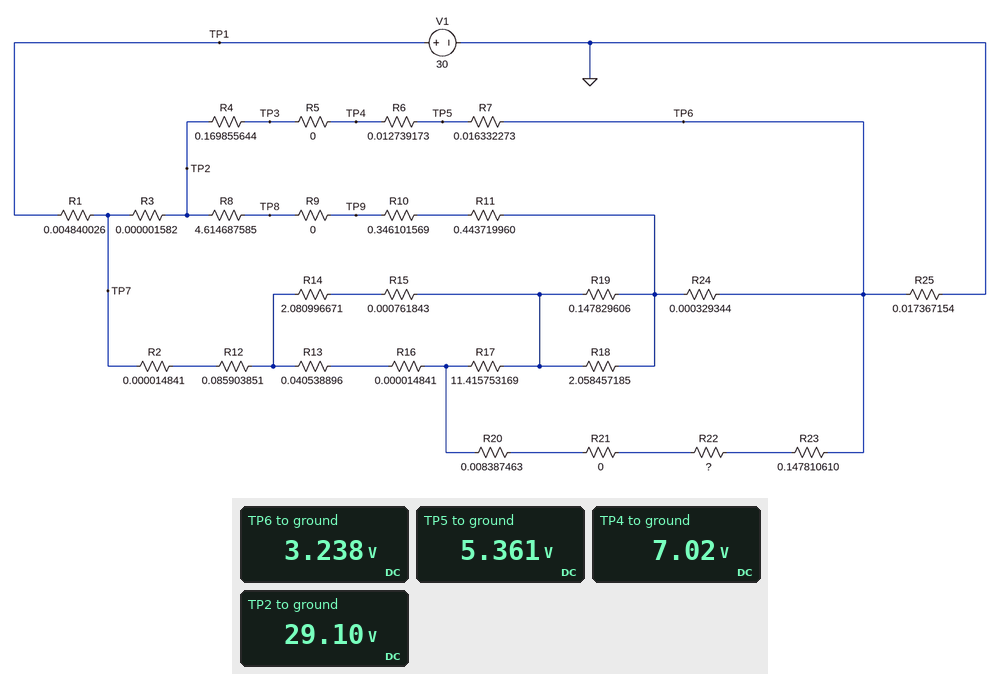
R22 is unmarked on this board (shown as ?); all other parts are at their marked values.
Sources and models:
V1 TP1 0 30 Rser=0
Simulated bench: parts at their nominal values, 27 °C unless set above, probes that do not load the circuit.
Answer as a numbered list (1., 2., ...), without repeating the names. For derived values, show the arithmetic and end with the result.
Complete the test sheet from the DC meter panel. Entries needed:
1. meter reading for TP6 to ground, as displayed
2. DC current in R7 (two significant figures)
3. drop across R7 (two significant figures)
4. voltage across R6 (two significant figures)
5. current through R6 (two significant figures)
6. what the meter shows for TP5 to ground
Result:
1. 3.238 V
2. (5.361 V - 3.238 V) / 16.33 mΩ = 130 A
3. 5.361 V - 3.238 V = 2.1 V
4. 7.02 V - 5.361 V = 1.7 V
5. (7.02 V - 5.361 V) / 12.74 mΩ = 130 A
6. 5.361 V
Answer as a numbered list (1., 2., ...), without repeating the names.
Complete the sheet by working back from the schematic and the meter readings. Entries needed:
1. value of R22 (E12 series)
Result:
1. 0.33 Ω
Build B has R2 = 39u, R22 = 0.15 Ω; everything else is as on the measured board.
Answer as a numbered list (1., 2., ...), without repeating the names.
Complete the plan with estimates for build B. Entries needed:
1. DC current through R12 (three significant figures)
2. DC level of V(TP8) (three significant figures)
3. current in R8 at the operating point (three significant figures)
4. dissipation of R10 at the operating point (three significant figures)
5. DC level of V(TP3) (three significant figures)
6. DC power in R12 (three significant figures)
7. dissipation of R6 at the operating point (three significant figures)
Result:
1. 67.1 A
2. 7.22 V
3. 4.73 A
4. 7.74 W
5. 7.21 V
6. 387 W
7. 210 W
